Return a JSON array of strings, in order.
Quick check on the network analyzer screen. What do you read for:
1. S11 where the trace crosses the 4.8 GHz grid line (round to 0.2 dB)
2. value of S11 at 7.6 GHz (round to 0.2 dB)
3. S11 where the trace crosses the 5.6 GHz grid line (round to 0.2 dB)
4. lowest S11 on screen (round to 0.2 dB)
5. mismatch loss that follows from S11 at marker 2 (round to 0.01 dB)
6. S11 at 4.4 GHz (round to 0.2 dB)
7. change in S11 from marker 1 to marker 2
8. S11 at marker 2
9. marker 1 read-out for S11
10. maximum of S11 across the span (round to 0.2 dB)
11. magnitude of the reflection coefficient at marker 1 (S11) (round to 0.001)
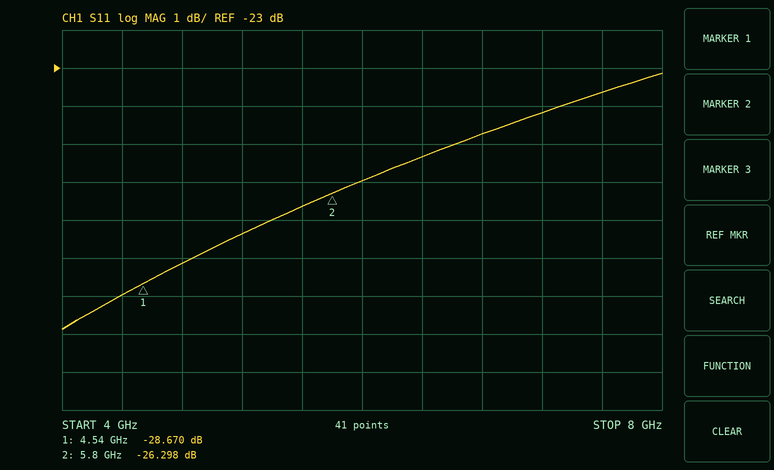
["-28.2 dB", "-23.6 dB", "-26.6 dB", "-29.8 dB", "0.01 dB", "-29.0 dB", "2.372 dB", "-26.298 dB", "-28.670 dB", "-23.2 dB", "0.037"]
